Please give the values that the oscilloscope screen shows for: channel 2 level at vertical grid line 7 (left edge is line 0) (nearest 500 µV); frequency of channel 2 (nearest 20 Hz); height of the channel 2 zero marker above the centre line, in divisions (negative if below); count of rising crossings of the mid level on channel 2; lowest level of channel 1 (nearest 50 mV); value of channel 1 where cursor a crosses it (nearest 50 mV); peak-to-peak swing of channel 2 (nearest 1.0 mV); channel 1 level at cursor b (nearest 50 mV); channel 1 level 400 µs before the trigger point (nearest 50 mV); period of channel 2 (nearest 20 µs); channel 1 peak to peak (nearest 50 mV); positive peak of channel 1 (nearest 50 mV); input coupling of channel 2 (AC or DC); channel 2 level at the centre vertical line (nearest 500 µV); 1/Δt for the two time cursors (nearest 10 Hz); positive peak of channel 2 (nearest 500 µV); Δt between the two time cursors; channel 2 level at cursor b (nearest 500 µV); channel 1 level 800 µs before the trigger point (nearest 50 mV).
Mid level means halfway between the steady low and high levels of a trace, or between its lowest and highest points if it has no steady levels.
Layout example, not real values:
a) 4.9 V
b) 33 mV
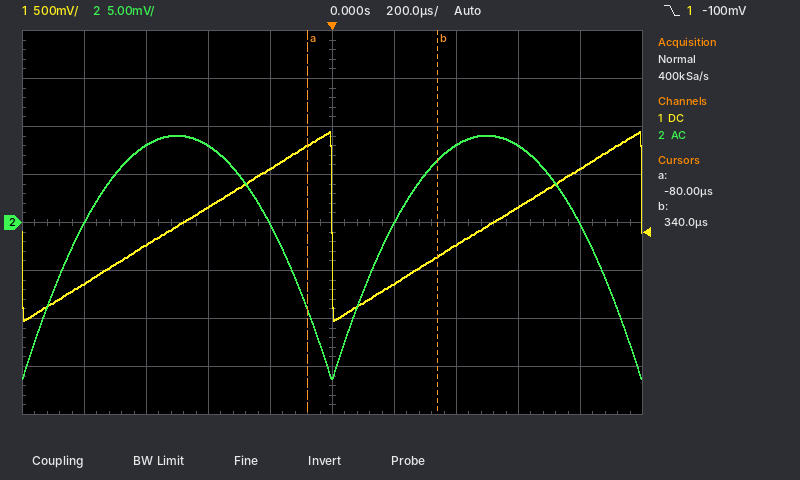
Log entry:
a) 8.0 mV
b) 1.00 kHz
c) 0.0 div
d) 2
e) -1.00 V
f) 800 mV
g) 25.0 mV
h) -350 mV
i) 150 mV
j) 1.00 ms
k) 1.95 V
l) 950 mV
m) AC
n) -16.0 mV
o) 2.38 kHz
p) 9.0 mV
q) 420 µs
r) 6.5 mV
s) -650 mV
